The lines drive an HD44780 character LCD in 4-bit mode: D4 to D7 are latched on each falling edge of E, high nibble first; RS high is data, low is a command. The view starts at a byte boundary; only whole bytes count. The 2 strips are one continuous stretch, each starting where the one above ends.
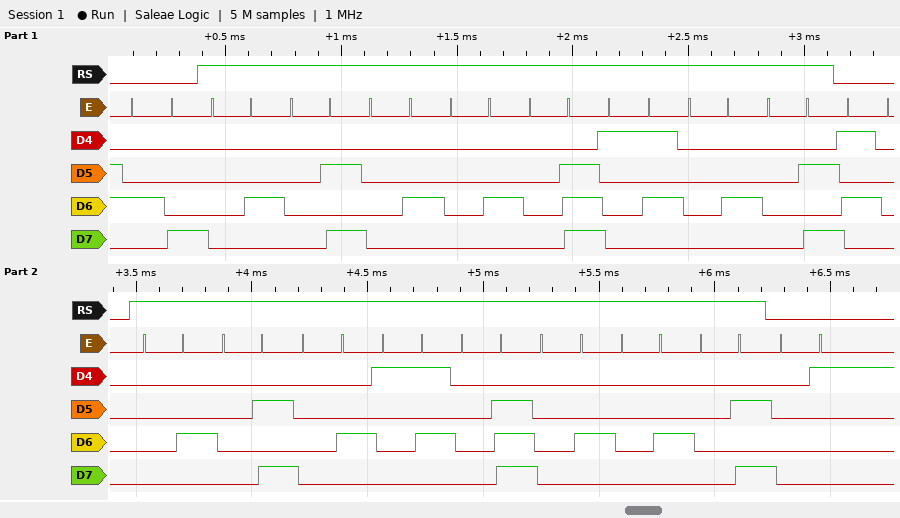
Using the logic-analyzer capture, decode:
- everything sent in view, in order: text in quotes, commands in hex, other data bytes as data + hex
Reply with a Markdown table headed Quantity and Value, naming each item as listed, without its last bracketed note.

| Quantity | Value |
|---|---|
| everything sent in view, in order: text in quotes, commands in hex, other data bytes as data + hex | 0x48 data 04 0A 04 04 0E 15 04 0A 0x50 data 04 0A 04 15 0E 04 04 0A 0x01 |
